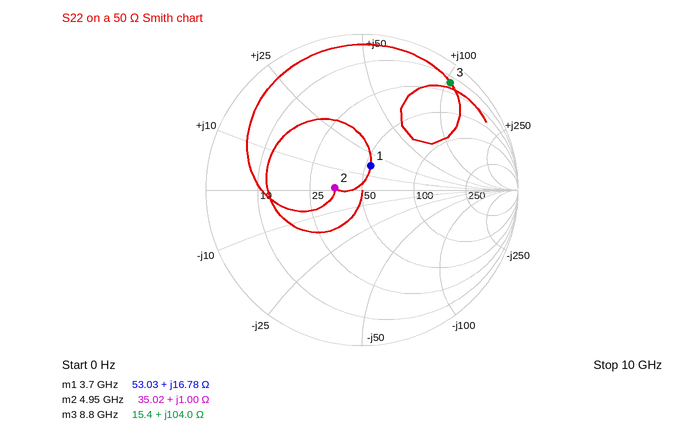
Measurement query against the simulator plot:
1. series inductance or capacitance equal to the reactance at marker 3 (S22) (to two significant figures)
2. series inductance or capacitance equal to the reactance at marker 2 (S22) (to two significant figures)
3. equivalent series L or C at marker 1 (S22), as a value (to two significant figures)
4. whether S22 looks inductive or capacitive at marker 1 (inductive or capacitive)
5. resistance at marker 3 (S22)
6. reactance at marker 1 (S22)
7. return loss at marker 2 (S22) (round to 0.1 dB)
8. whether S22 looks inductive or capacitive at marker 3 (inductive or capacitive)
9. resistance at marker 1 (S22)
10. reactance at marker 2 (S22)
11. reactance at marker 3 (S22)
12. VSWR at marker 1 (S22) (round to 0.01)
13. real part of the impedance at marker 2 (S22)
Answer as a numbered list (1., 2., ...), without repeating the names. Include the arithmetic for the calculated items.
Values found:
1. L = 104 Ω/(2π × 8.8 GHz) ≈ 1.9 nH
2. L = 1 Ω/(2π × 4.95 GHz) ≈ 32 pH
3. L = 16.78 Ω/(2π × 3.7 GHz) ≈ 722 pH, so 720 pH to two significant figures
4. inductive
5. 15.4 Ω
6. +16.78 Ω
7. 15.1 dB
8. inductive
9. 53.03 Ω
10. +1.00 Ω
11. +104.0 Ω
12. 1.39
13. 35.02 Ω
